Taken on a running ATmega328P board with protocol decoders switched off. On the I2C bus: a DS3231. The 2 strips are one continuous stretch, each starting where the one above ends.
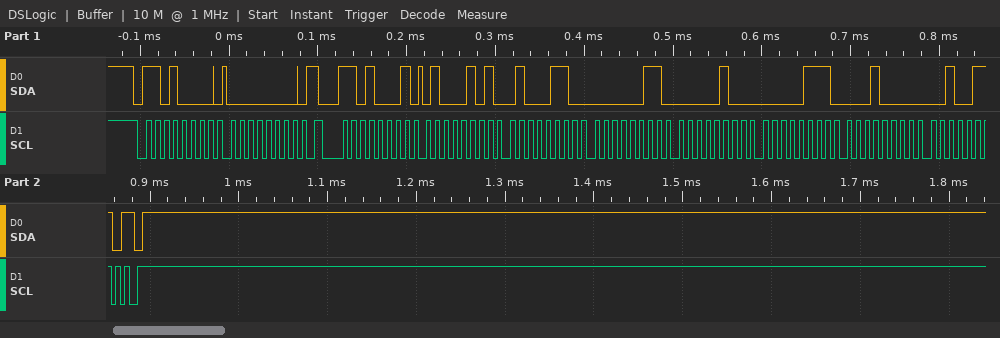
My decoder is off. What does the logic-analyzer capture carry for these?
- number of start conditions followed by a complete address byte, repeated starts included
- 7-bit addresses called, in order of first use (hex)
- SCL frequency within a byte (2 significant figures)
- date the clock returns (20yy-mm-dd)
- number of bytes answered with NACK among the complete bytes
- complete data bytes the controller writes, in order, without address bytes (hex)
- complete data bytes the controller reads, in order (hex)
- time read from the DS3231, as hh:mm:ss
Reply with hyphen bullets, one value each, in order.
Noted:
- 2
- 0x68
- 100 kHz
- 2026-10-07
- 1
- 00
- 45 46 03 04 07 10 26
- 03:46:45
